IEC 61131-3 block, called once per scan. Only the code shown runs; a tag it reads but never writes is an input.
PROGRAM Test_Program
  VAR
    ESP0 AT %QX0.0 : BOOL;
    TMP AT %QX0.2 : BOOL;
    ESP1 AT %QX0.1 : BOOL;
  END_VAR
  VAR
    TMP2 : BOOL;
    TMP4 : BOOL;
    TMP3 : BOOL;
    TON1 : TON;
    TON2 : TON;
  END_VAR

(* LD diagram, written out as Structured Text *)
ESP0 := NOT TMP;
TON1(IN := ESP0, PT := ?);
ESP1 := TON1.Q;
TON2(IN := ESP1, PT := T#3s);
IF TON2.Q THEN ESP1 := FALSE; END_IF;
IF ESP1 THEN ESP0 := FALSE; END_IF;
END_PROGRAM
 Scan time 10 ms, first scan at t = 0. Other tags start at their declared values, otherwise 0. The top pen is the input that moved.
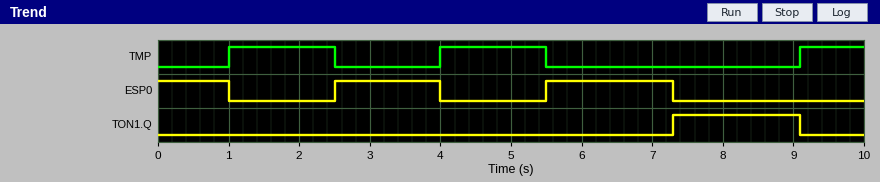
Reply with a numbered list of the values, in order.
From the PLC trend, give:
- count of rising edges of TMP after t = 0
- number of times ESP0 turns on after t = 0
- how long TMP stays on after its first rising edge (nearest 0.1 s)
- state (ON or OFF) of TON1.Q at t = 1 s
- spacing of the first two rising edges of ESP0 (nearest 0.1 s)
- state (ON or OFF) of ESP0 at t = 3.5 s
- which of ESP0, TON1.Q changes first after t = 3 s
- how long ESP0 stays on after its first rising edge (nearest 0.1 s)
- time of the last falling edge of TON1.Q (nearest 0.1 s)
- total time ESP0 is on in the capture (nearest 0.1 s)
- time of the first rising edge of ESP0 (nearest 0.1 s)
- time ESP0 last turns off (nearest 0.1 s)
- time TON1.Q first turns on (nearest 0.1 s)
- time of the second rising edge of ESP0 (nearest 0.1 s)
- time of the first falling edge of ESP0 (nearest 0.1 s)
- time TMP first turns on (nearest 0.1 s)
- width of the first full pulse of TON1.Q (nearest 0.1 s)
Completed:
1. 3
2. 2
3. 1.5 s
4. OFF
5. 3.0 s
6. ON
7. ESP0
8. 1.5 s
9. 9.1 s
10. 4.3 s
11. 2.5 s
12. 7.3 s
13. 7.3 s
14. 5.5 s
15. 1.0 s
16. 1.0 s
17. 1.8 s
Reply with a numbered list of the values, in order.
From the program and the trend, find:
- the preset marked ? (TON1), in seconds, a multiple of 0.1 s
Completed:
1. 1.8 s
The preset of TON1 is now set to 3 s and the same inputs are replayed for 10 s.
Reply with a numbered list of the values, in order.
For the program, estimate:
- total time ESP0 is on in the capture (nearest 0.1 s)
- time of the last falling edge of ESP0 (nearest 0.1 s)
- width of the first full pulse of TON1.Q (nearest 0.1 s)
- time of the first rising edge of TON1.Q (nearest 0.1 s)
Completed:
1. 5.5 s
2. 8.5 s
3. 0.6 s
4. 8.5 s
